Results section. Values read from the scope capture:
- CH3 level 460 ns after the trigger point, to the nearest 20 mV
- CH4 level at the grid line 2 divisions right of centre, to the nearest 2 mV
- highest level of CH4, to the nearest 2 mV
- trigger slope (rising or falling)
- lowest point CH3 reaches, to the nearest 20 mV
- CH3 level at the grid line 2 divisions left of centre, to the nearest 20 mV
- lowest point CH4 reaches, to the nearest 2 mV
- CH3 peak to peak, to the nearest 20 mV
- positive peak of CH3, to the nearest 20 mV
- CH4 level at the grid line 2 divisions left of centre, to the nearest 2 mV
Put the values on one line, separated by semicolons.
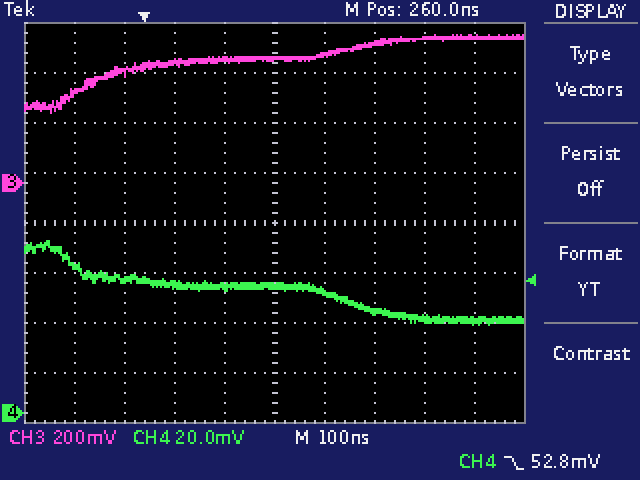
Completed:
560 mV; 40 mV; 68 mV; falling; 280 mV; 480 mV; 36 mV; 320 mV; 600 mV; 52 mV
